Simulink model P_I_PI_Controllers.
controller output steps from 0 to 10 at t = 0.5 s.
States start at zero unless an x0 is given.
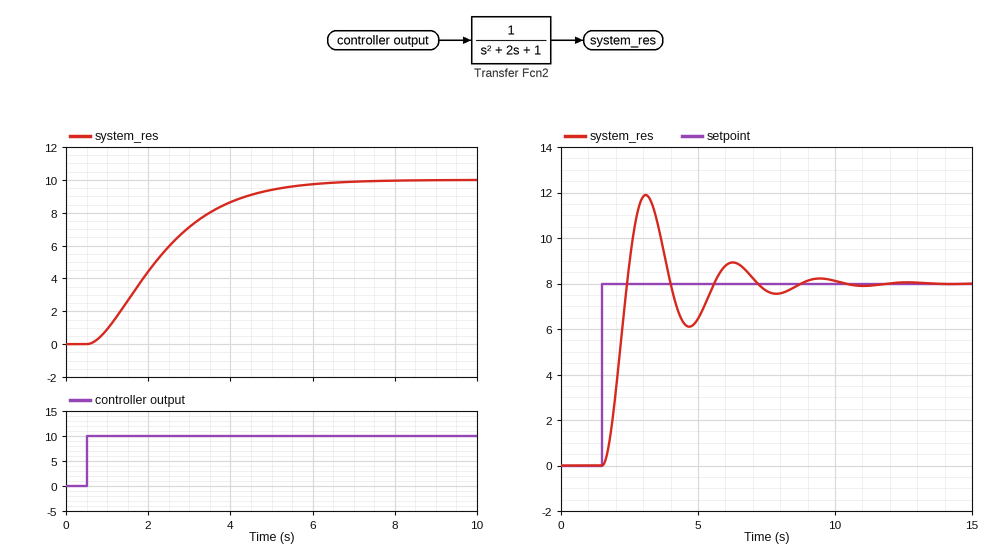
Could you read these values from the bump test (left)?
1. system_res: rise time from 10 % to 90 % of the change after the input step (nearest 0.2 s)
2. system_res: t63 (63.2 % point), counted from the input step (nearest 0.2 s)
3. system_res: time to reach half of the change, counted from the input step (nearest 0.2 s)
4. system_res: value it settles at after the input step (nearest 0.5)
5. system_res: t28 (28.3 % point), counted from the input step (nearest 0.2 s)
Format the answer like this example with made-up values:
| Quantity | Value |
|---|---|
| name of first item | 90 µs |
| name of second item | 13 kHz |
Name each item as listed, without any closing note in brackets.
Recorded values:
| Quantity | Value |
|---|---|
| system_res: rise time from 10 % to 90 % of the change after the input step | 3.4 s |
| system_res: t63 (63.2 % point), counted from the input step | 2.2 s |
| system_res: time to reach half of the change, counted from the input step | 1.6 s |
| system_res: value it settles at after the input step | 10.0 |
| system_res: t28 (28.3 % point), counted from the input step | 1.0 s |
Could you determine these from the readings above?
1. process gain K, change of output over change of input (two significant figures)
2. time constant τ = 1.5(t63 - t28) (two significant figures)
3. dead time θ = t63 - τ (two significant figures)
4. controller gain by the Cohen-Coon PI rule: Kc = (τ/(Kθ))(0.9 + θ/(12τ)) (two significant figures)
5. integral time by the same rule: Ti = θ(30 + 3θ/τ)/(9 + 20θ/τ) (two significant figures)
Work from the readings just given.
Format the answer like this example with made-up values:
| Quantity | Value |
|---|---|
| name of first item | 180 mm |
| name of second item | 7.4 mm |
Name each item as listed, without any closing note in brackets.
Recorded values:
| Quantity | Value |
|---|---|
| process gain K, change of output over change of input | 1.0 |
| time constant τ = 1.5(t63 - t28) | 1.8 s |
| dead time θ = t63 - τ | 0.40 s |
| controller gain by the Cohen-Coon PI rule: Kc = (τ/(Kθ))(0.9 + θ/(12τ)) | 4.1 |
| integral time by the same rule: Ti = θ(30 + 3θ/τ)/(9 + 20θ/τ) | 0.91 s |
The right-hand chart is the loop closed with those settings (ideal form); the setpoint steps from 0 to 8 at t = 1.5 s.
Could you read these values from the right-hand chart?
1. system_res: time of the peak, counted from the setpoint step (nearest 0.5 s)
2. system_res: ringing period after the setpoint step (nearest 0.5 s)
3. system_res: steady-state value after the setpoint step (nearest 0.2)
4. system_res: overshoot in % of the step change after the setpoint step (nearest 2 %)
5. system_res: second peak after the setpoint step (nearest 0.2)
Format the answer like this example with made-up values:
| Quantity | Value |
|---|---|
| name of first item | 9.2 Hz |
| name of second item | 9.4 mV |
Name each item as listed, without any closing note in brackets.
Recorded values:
| Quantity | Value |
|---|---|
| system_res: time of the peak, counted from the setpoint step | 1.5 s |
| system_res: ringing period after the setpoint step | 3.0 s |
| system_res: steady-state value after the setpoint step | 8.0 |
| system_res: overshoot in % of the step change after the setpoint step | 48 % |
| system_res: second peak after the setpoint step | 9.0 |
